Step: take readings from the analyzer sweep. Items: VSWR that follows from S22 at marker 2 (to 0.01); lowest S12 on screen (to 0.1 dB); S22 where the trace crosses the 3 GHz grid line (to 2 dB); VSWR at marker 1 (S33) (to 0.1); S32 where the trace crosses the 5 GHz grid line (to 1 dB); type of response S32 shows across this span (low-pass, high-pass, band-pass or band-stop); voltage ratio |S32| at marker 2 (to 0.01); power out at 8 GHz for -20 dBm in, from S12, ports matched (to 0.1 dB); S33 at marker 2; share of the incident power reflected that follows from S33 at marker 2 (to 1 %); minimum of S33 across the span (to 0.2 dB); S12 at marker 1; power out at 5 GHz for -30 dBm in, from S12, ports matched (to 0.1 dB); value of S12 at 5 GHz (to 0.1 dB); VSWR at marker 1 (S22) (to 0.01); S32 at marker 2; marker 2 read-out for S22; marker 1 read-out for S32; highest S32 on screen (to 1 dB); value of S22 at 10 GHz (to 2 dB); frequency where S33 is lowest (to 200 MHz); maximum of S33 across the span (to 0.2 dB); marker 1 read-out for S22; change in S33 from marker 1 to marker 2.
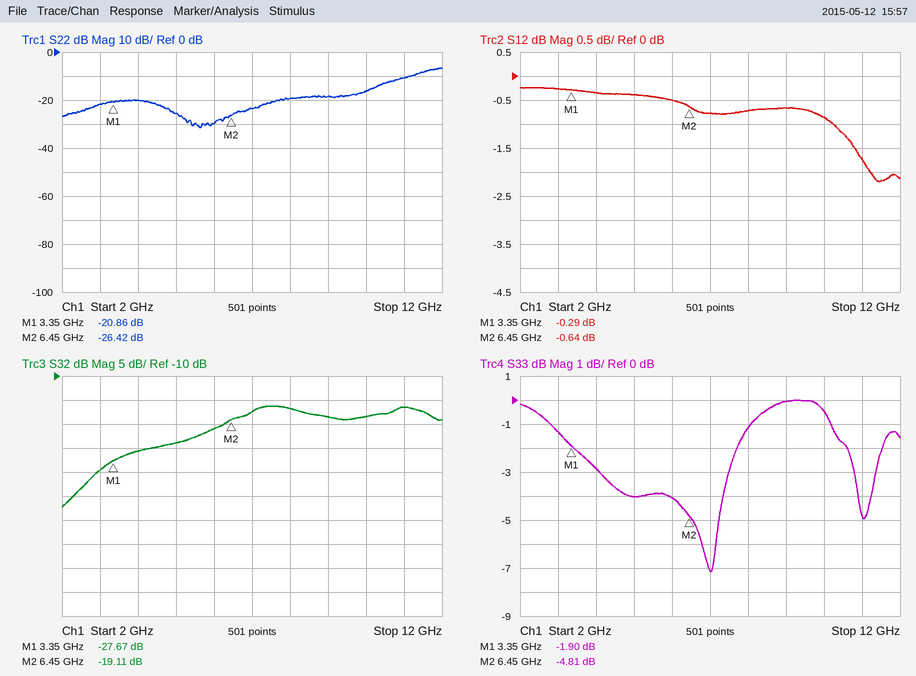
1.10
-2.2 dB
-22 dB
9.2
-24 dB
high-pass
0.11
-20.7 dBm
-4.81 dB
33 %
-7.2 dB
-0.29 dB
-30.4 dBm
-0.4 dB
1.20
-19.11 dB
-26.42 dB
-27.67 dB
-16 dB
-16 dB
7.0 GHz
0.0 dB
-20.86 dB
-2.91 dB
